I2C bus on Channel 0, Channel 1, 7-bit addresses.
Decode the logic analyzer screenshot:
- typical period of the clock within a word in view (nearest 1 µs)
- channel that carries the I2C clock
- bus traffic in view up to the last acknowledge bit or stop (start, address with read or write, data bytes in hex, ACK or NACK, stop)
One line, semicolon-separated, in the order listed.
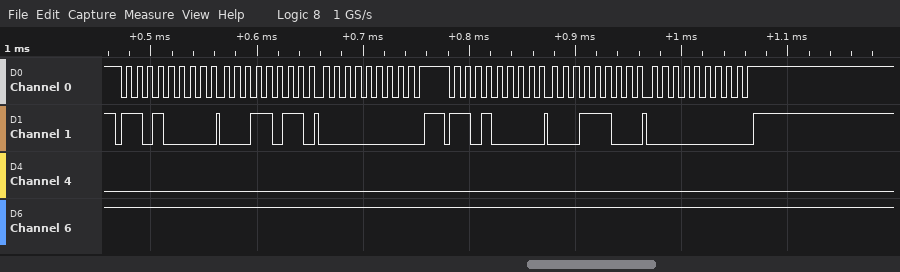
10 µs; Channel 0; start, address 68 write ACK, 1B ACK, 00 ACK, stop, start, address 68 write ACK, 1C ACK, 00 ACK, stop
